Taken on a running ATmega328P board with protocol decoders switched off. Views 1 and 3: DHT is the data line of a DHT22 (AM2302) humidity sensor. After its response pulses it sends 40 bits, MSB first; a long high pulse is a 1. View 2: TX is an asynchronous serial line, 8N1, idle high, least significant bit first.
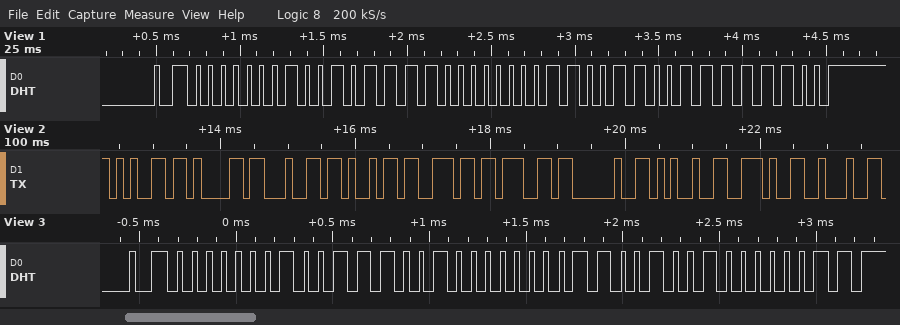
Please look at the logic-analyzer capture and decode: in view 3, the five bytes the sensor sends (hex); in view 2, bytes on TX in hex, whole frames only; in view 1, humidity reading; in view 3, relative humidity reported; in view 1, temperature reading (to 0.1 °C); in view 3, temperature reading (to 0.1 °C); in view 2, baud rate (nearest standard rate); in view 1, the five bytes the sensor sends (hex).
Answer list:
01 39 00 C9 03
0x65 0x61 0x64 0x69 0x6E 0x67 0x20 0x25 0x2E 0x22
30.3 %
31.3 %
20.4 °C
20.1 °C
9600 baud
01 2F 00 CC FC
